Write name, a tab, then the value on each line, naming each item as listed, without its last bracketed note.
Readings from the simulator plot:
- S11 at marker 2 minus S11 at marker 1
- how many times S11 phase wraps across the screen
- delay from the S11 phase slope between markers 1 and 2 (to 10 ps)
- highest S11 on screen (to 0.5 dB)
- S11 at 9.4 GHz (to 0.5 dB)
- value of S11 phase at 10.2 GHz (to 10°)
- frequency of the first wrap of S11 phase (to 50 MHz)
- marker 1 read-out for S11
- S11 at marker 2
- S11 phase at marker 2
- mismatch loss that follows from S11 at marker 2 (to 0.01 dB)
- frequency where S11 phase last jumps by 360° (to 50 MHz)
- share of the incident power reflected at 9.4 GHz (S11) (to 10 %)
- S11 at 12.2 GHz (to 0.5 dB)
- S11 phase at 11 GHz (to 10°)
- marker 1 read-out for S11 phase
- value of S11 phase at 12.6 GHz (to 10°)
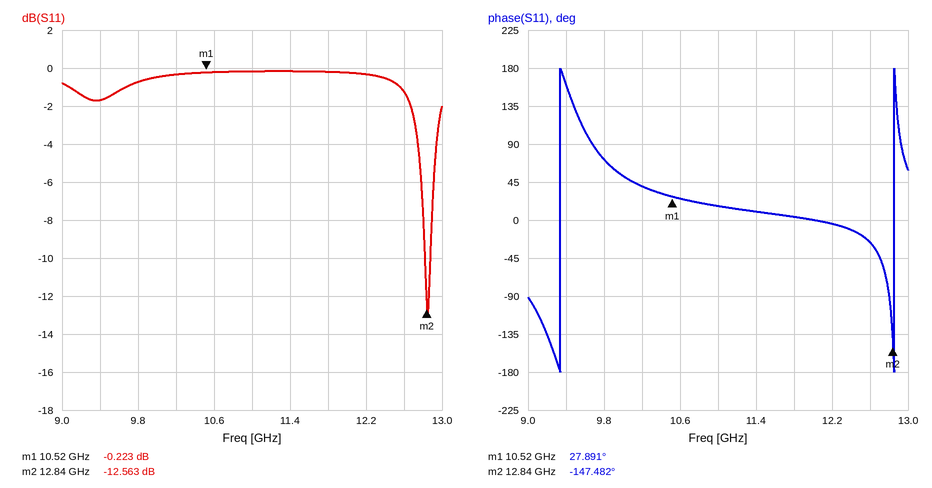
S11 at marker 2 minus S11 at marker 1	-12.340 dB
how many times S11 phase wraps across the screen	2
delay from the S11 phase slope between markers 1 and 2	210 ps
highest S11 on screen	0.0 dB
S11 at 9.4 GHz	-1.5 dB
value of S11 phase at 10.2 GHz	40°
frequency of the first wrap of S11 phase	9.35 GHz
marker 1 read-out for S11	-0.223 dB
S11 at marker 2	-12.563 dB
S11 phase at marker 2	-147.482°
mismatch loss that follows from S11 at marker 2	0.25 dB
frequency where S11 phase last jumps by 360°	12.85 GHz
share of the incident power reflected at 9.4 GHz (S11)	70 %
S11 at 12.2 GHz	-0.5 dB
S11 phase at 11 GHz	20°
marker 1 read-out for S11 phase	27.891°
value of S11 phase at 12.6 GHz	-30°
